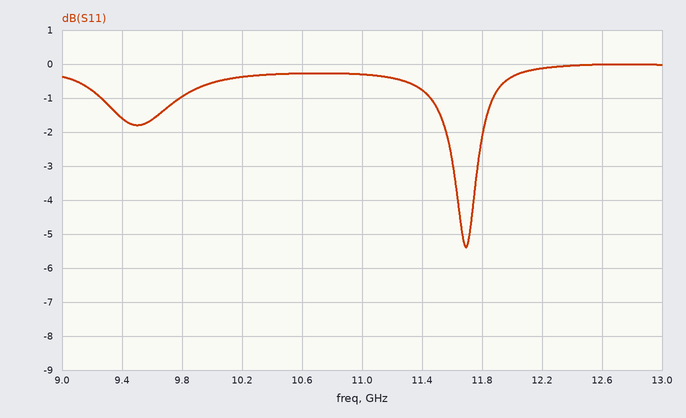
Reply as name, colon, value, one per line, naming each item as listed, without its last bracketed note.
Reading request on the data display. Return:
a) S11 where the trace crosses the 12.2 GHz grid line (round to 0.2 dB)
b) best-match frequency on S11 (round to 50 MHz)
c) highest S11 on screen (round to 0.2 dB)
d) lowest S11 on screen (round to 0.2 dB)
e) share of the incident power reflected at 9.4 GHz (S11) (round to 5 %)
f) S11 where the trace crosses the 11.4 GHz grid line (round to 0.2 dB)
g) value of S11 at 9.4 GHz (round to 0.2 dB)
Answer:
S11 where the trace crosses the 12.2 GHz grid line: -0.2 dB
best-match frequency on S11: 11.70 GHz
highest S11 on screen: 0.0 dB
lowest S11 on screen: -5.4 dB
share of the incident power reflected at 9.4 GHz (S11): 70 %
S11 where the trace crosses the 11.4 GHz grid line: -0.8 dB
value of S11 at 9.4 GHz: -1.6 dB
